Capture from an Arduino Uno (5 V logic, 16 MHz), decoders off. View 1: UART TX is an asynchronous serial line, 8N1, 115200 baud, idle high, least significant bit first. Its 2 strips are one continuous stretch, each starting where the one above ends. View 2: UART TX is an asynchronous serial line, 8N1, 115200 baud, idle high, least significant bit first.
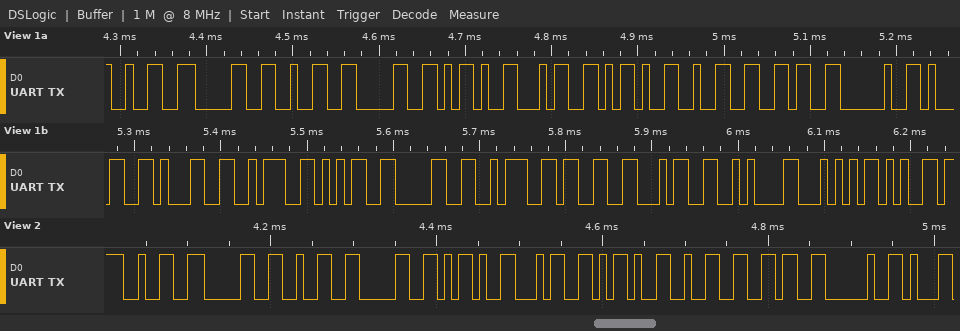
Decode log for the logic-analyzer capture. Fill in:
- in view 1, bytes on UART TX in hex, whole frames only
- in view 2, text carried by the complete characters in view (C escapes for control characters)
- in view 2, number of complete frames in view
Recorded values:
0x32 0x30 0x32 0x30 0x2D 0x34 0x2D 0x32 0x36 0x20 0x31 0x31 0x3A 0x35 0x30 0x3A 0x33 0x34 0x0A 0x54 0x65
"2020-4-26 "
10
